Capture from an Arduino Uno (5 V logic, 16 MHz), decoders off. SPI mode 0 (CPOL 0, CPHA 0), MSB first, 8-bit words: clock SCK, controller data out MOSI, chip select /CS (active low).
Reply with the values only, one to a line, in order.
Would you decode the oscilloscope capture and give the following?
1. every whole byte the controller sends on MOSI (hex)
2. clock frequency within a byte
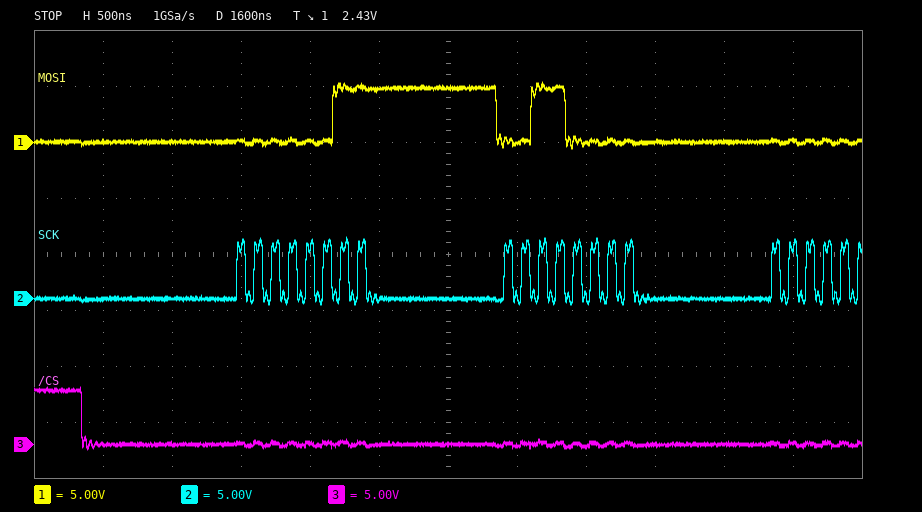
03 30
8 MHz
